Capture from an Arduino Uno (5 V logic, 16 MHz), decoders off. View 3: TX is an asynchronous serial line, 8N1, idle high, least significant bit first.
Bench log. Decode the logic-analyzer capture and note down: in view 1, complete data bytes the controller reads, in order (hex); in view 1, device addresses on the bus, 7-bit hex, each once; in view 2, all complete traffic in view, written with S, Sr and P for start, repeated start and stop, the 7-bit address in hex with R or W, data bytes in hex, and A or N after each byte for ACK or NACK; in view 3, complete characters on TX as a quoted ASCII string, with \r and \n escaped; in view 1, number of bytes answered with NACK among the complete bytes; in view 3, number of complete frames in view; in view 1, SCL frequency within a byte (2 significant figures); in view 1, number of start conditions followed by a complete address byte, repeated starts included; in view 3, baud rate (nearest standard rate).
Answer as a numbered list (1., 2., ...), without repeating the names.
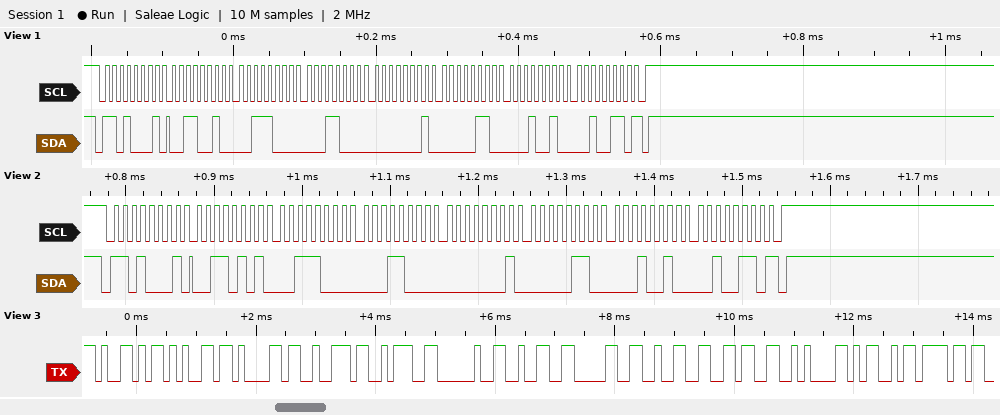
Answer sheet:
1. 32 38 18 01 06 12 26
2. 0x68
3. S 68R A 35 A 38 A 18 A 01 A 06 A 12 A 26 N P
4. "Year: 2026\nMo"
5. 1
6. 13
7. 100 kHz
8. 1
9. 9600 baud
